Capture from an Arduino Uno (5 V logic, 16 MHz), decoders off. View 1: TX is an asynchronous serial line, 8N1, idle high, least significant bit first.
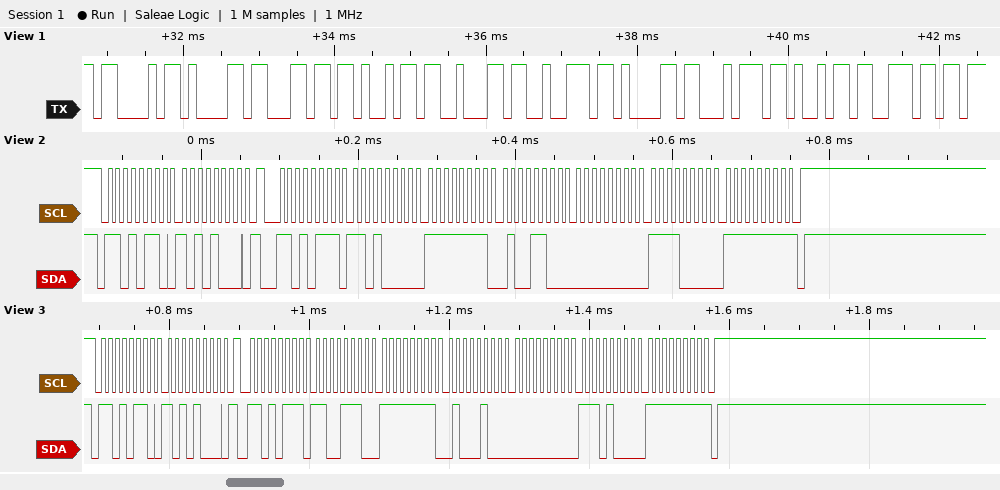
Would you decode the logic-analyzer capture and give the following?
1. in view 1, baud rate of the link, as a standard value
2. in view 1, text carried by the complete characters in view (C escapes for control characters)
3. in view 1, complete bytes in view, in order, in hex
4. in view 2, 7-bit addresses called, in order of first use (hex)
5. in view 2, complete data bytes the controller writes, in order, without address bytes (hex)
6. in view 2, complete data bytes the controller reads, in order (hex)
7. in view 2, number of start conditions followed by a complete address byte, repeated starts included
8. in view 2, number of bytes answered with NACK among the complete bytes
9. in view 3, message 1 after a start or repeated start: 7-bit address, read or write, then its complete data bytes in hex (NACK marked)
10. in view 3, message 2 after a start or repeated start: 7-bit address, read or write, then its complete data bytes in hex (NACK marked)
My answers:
9600 baud
"Calibratin"
0x43 0x61 0x6C 0x69 0x62 0x72 0x61 0x74 0x69 0x6E
0x6B
A8
D0 FF 4C 00 F0 FF
2
1
0x6B write: A8
0x6B read: CE FF 44 00 E8 FF NACK
